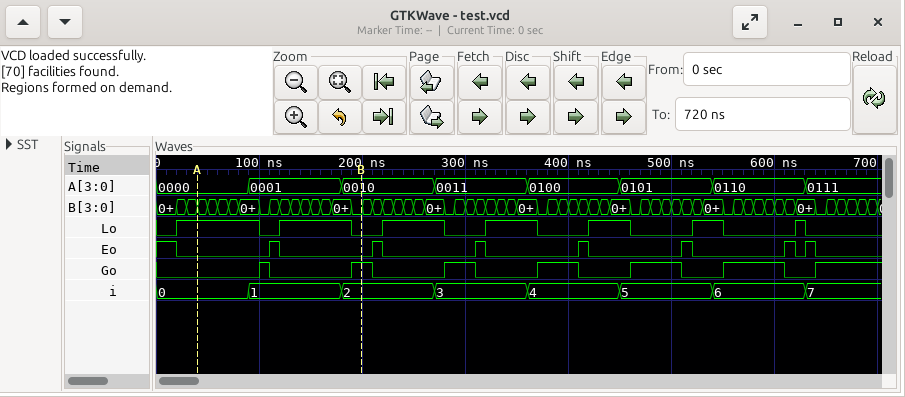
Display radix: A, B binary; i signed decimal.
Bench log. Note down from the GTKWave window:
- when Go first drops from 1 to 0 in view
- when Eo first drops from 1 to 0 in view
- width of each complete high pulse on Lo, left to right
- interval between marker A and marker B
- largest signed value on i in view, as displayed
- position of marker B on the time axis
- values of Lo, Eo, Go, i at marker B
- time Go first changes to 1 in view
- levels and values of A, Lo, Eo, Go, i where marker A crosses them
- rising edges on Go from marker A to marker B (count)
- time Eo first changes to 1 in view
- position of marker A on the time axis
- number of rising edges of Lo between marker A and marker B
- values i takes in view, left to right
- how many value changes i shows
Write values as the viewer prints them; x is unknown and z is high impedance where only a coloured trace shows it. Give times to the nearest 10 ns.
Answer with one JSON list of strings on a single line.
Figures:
["110 ns", "20 ns", "80 ns, 70 ns, 60 ns, 50 ns, 40 ns, 30 ns, 10 ns", "160 ns", "7", "200 ns", "Lo=0, Eo=0, Go=1, i=2", "100 ns", "A=0000, Lo=1, Eo=0, Go=0, i=0", "2", "110 ns", "40 ns", "1", "0, 1, 2, 3, 4, 5, 6, 7", "7"]
